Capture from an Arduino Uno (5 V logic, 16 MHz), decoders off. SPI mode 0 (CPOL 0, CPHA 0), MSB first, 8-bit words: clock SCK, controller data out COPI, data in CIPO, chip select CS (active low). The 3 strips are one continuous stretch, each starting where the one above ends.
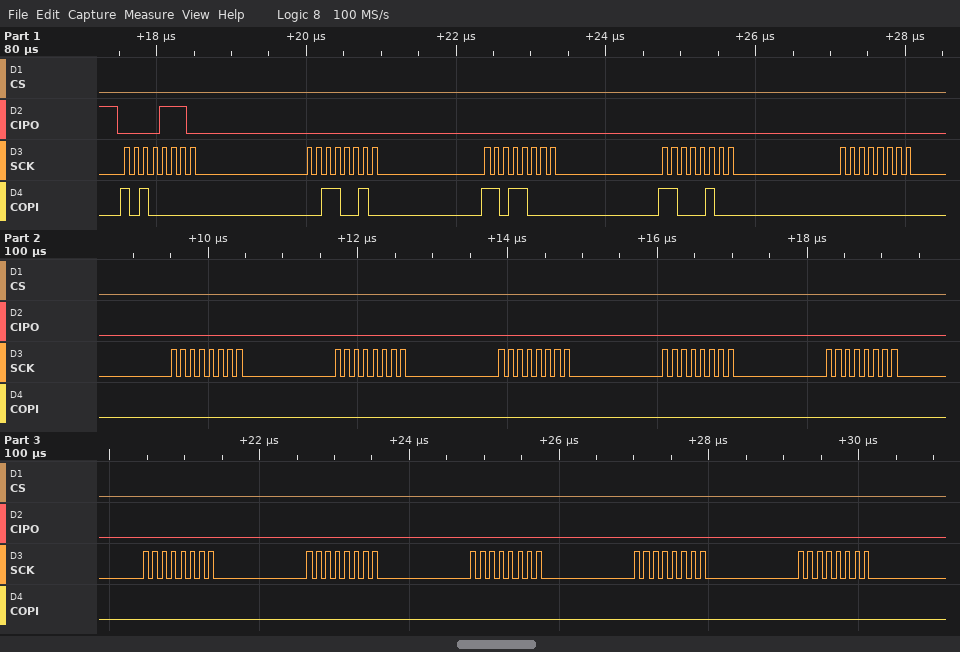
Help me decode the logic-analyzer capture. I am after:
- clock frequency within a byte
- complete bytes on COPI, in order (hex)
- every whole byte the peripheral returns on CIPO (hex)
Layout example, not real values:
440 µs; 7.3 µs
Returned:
8 MHz; A0 32 D8 C4 00 00 00 00 00 00 00 00 00 00 00; 0E 00 00 00 00 00 00 00 00 00 00 00 00 00 00
